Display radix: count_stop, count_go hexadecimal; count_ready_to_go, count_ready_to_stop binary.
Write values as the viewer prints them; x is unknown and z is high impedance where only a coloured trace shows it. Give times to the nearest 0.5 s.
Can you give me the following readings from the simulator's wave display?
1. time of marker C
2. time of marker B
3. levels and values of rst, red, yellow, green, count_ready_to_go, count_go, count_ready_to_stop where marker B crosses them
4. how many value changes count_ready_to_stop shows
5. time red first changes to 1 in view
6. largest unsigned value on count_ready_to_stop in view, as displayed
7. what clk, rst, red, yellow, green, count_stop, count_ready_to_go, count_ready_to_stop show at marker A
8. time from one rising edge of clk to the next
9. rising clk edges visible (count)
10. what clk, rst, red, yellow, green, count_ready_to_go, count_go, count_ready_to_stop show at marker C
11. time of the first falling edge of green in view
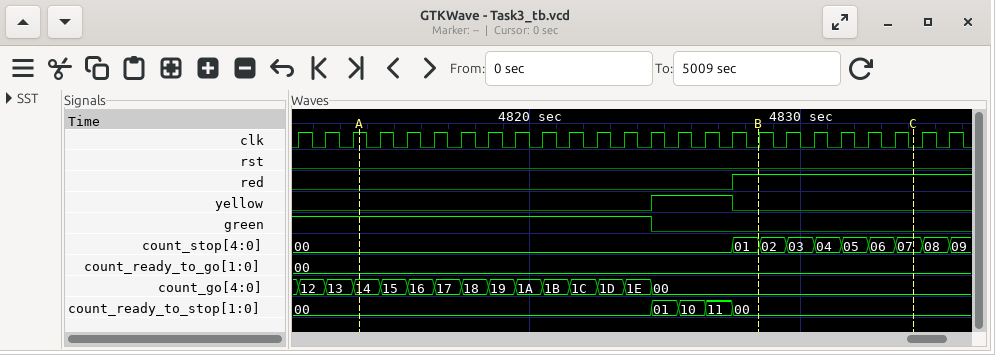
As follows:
4834 s
4828.5 s
rst=0, red=1, yellow=0, green=0, count_ready_to_go=00, count_go=00, count_ready_to_stop=00
4
4827.5 s
11
clk=1, rst=0, red=0, yellow=0, green=1, count_stop=00, count_ready_to_go=00, count_ready_to_stop=00
1 s
25
clk=0, rst=0, red=1, yellow=0, green=0, count_ready_to_go=00, count_go=00, count_ready_to_stop=00
4824.5 s
